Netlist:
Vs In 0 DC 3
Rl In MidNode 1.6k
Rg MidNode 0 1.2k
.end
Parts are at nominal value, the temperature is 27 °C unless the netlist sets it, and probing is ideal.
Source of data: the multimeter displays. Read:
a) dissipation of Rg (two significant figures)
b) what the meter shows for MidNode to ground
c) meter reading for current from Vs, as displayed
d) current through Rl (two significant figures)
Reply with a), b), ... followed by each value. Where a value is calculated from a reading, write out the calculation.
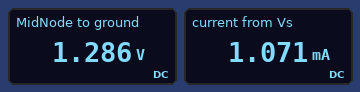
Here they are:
a) (1.286 V)^2 / 1.2 kΩ = 1.4 mW
b) 1.286 V
c) 1.071 mA
d) (3 V - 1.286 V) / 1.6 kΩ = 1.1 mA
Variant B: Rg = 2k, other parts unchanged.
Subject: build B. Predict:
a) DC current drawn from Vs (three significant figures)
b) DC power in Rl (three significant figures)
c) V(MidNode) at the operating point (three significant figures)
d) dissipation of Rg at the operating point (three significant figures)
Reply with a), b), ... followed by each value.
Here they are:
a) 833 µA
b) 1.11 mW
c) 1.67 V
d) 1.39 mW
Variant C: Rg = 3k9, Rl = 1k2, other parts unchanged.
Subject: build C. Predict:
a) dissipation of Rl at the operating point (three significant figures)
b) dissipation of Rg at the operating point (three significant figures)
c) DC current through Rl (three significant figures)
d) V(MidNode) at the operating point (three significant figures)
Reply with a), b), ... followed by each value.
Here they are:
a) 415 µW
b) 1.35 mW
c) 588 µA
d) 2.29 V
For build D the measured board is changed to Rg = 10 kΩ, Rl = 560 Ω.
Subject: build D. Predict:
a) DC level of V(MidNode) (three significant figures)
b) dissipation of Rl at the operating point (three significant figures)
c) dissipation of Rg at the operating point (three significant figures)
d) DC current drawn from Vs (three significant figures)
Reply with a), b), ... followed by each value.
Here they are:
a) 2.84 V
b) 45.2 µW
c) 807 µW
d) 284 µA
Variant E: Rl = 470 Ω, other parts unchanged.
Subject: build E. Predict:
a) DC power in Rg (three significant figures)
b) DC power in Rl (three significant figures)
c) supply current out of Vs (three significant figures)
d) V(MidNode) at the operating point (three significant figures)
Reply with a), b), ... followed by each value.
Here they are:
a) 3.87 mW
b) 1.52 mW
c) 1.80 mA
d) 2.16 V
